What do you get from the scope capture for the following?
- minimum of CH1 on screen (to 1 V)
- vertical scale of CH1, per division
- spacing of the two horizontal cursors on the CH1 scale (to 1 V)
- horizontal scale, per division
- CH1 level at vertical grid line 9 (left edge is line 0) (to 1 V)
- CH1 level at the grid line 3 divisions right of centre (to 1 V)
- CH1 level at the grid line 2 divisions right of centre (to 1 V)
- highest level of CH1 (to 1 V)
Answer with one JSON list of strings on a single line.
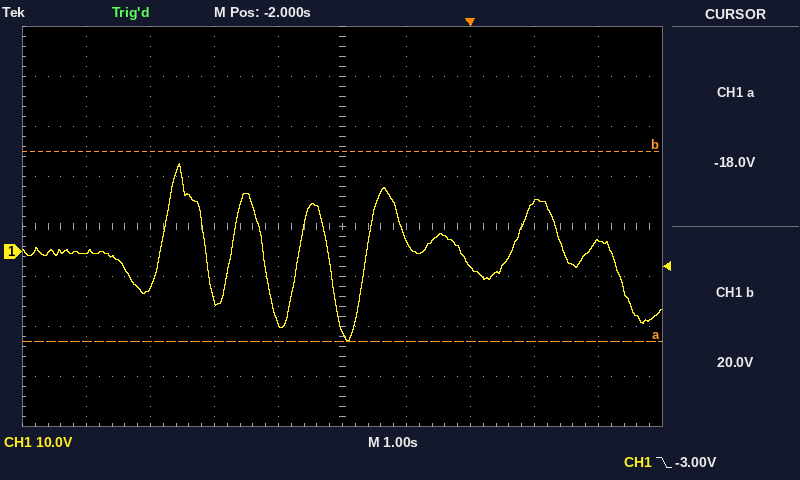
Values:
["-18 V", "10 V", "38 V", "1 s", "2 V", "10 V", "-3 V", "18 V"]
